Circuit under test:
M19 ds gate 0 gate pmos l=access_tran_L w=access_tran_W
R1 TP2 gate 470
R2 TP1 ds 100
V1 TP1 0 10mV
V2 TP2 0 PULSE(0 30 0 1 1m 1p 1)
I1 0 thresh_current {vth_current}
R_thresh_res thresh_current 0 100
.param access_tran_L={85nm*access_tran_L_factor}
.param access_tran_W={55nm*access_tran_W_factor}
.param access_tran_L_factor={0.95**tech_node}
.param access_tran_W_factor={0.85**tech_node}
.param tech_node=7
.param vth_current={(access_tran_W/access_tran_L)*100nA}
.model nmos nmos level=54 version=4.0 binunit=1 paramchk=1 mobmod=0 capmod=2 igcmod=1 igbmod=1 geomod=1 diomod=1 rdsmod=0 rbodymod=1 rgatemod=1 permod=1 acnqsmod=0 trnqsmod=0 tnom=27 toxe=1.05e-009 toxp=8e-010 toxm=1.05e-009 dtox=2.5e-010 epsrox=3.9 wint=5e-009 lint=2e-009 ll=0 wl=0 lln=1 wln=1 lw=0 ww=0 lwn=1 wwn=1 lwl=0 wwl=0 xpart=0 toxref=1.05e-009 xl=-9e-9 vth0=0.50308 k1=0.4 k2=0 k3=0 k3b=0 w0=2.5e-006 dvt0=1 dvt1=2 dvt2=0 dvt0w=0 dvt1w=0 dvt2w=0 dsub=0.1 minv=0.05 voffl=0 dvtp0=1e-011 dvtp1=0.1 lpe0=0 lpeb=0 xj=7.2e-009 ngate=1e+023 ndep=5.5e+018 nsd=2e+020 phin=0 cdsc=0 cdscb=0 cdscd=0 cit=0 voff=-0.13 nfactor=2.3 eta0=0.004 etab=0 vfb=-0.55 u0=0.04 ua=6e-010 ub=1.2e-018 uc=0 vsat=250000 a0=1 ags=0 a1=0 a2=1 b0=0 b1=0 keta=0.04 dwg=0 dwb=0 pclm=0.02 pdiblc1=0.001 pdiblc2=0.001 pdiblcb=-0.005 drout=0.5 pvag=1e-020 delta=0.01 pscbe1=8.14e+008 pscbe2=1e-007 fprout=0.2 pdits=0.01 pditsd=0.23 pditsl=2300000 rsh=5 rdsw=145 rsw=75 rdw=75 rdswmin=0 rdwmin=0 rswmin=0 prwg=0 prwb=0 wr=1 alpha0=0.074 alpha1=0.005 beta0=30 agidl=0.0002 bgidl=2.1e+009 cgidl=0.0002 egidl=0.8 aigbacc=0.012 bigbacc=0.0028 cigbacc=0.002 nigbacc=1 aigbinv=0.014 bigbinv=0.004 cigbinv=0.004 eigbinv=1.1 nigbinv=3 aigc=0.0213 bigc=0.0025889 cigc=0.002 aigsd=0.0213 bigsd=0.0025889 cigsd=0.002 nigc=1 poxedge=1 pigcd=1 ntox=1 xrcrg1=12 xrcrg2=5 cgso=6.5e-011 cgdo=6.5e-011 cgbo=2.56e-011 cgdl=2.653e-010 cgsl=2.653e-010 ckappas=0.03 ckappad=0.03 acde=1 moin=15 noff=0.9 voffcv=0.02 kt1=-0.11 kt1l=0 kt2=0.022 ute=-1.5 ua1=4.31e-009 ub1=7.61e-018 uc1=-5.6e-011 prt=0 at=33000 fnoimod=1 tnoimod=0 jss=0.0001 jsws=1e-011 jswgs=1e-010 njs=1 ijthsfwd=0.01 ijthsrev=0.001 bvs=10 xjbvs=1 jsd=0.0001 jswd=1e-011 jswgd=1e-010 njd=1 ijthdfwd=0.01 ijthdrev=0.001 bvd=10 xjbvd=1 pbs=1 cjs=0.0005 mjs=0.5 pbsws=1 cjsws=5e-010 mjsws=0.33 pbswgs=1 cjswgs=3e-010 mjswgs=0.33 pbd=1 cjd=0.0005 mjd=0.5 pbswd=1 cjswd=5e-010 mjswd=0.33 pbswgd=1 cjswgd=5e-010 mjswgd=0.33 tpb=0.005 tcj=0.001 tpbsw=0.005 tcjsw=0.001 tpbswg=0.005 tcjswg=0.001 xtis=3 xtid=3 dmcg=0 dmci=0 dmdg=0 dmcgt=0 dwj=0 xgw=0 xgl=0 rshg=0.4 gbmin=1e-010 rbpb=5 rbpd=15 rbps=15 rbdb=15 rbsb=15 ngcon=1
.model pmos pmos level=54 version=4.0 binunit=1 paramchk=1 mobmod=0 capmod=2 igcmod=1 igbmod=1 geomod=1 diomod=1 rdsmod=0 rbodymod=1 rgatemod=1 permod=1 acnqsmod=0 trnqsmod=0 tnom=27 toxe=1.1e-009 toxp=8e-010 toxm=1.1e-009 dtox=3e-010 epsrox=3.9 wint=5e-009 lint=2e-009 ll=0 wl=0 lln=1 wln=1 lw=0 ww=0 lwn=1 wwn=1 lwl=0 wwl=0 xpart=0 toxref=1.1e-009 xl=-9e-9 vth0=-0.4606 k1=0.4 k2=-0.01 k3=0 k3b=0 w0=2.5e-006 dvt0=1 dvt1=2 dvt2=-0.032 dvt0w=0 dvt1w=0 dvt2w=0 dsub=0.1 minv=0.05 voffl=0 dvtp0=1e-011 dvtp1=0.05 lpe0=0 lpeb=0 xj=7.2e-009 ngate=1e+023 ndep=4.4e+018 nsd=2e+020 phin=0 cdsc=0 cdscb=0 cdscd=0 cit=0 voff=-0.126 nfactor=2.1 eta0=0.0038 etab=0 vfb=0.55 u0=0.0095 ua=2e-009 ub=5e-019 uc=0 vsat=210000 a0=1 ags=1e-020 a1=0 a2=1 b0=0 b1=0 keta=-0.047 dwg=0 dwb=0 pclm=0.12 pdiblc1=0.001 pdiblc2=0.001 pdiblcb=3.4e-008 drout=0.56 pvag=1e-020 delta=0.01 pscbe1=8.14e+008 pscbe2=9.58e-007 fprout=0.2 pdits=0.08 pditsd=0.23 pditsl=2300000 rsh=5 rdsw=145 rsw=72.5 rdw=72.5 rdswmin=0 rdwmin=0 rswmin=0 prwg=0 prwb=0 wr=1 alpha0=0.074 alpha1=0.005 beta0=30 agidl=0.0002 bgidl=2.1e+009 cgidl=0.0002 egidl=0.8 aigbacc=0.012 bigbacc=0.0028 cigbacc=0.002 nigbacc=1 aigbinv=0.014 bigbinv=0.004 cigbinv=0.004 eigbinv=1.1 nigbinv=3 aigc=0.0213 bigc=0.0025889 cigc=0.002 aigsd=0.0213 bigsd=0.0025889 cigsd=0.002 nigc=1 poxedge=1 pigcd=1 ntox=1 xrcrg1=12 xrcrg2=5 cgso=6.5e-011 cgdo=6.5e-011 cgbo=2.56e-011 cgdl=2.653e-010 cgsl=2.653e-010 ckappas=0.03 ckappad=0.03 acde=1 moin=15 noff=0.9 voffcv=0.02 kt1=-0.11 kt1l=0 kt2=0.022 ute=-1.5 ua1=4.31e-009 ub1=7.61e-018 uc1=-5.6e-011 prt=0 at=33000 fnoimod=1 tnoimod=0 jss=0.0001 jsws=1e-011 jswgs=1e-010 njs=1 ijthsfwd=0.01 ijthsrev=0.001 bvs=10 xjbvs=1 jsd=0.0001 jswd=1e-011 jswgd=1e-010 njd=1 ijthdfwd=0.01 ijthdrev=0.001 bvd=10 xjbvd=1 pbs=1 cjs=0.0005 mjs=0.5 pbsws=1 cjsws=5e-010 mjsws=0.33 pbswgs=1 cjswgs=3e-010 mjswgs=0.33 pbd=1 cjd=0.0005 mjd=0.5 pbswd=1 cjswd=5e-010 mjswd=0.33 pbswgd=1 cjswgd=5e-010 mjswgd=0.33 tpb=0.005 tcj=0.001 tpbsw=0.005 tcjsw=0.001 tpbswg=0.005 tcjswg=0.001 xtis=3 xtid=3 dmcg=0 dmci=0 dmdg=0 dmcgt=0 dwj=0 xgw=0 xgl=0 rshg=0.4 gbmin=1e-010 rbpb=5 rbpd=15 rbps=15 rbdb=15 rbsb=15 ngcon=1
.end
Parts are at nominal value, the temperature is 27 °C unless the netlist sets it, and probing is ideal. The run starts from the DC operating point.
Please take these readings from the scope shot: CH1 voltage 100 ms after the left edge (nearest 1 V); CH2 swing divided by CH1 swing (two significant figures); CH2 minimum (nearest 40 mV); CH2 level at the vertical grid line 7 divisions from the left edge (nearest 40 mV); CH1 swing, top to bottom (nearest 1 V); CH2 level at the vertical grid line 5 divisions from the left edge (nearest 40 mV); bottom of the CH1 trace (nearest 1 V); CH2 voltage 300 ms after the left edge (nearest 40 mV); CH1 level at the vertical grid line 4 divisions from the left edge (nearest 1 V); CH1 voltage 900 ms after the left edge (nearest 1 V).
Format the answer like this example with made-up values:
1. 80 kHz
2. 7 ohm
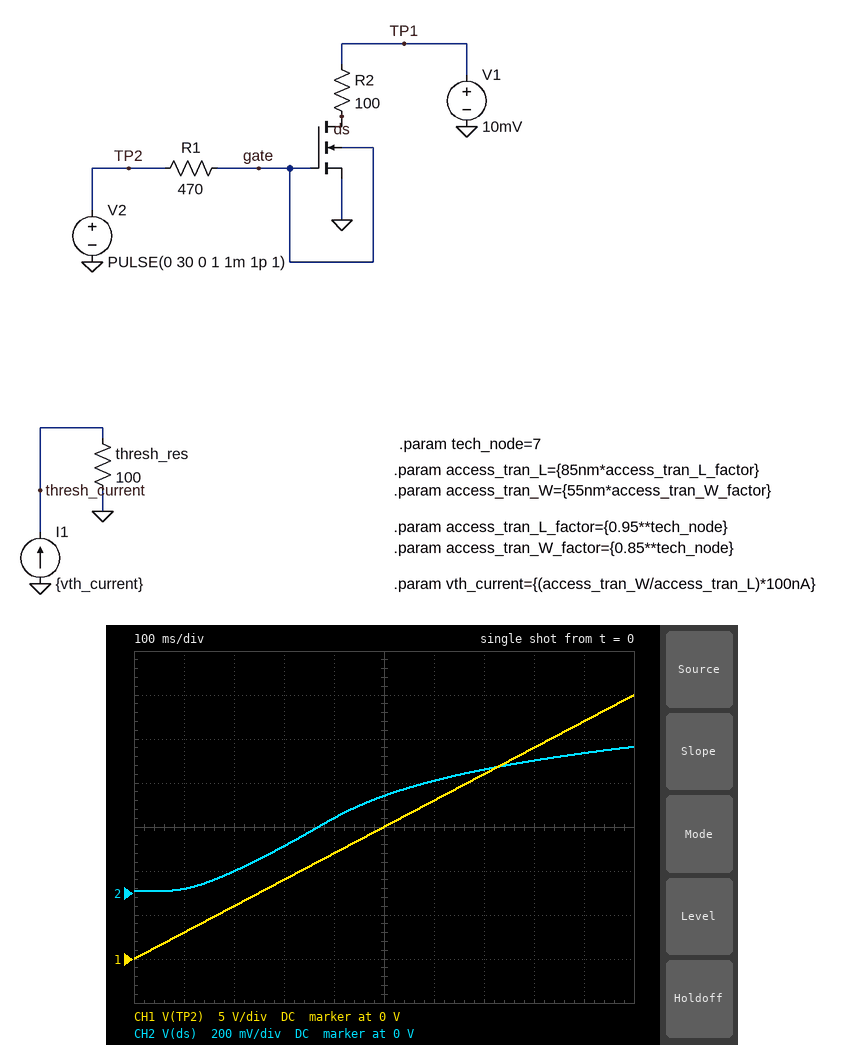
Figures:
1. 3 V
2. 0.022
3. 0 V
4. 560 mV
5. 30 V
6. 440 mV
7. 0 V
8. 200 mV
9. 12 V
10. 27 V
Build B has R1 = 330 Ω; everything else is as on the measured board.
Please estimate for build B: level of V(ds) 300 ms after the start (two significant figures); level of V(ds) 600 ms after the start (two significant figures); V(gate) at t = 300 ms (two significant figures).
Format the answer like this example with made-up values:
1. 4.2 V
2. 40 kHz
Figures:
1. 240 mV
2. 570 mV
3. 7.4 V
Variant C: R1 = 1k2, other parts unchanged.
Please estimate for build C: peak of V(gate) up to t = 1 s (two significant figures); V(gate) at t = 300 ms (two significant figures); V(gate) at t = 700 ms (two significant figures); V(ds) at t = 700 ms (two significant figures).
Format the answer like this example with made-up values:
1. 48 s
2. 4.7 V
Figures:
1. 9.0 V
2. 5.8 V
3. 8.7 V
4. 400 mV
